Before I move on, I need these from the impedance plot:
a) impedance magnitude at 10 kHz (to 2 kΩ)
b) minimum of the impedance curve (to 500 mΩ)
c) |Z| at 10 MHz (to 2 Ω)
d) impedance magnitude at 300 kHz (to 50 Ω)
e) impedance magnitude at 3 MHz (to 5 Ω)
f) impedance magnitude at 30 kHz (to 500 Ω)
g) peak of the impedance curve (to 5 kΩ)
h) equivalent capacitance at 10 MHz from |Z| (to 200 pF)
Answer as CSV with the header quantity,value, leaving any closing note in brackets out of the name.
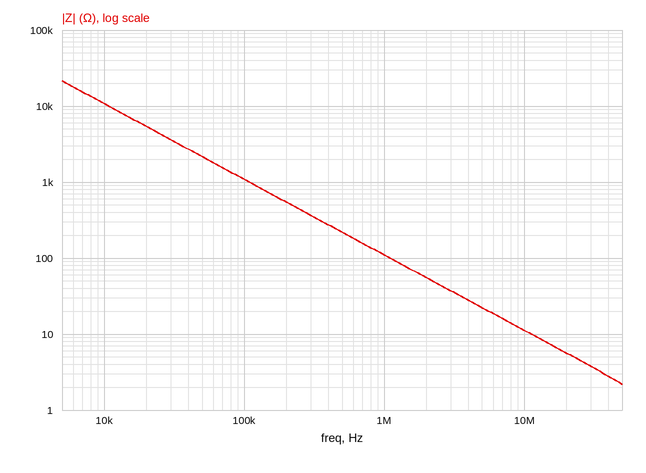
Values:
quantity,value
impedance magnitude at 10 kHz,10 kΩ
minimum of the impedance curve,2.0 Ω
|Z| at 10 MHz,12 Ω
impedance magnitude at 300 kHz,350 Ω
impedance magnitude at 3 MHz,35 Ω
impedance magnitude at 30 kHz,3.5 kΩ
peak of the impedance curve,20 kΩ
equivalent capacitance at 10 MHz from |Z|,1.4 nF
